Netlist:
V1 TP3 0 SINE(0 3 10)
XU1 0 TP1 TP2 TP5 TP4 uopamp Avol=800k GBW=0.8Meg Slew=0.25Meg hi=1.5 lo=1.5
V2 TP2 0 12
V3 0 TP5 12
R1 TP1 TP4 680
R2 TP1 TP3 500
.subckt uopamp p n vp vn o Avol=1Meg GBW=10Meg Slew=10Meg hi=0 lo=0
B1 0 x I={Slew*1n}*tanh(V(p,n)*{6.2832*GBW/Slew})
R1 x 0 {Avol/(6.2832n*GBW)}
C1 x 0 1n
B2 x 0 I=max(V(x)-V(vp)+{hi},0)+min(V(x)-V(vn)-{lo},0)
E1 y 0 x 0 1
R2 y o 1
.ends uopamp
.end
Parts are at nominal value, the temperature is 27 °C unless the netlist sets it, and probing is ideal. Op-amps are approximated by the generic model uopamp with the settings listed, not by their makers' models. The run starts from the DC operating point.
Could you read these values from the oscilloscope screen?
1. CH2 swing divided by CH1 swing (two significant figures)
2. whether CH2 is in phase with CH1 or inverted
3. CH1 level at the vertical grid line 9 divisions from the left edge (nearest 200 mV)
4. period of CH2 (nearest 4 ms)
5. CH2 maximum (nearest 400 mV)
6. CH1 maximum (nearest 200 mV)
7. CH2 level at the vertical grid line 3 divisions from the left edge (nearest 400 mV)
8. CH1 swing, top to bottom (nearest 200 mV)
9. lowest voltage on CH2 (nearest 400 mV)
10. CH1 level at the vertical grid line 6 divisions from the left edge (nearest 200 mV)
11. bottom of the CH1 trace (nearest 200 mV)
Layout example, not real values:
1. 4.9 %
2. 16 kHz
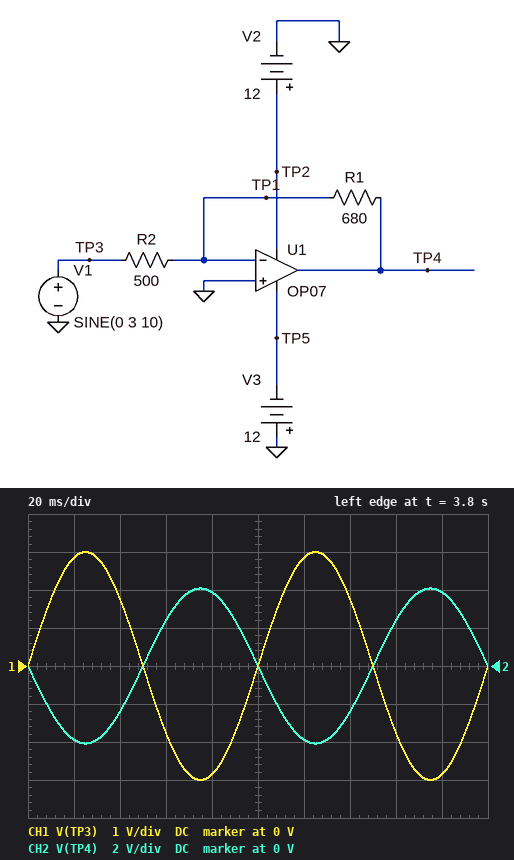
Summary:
1. 1.4
2. inverted
3. -2.8 V
4. 100 ms
5. 4.0 V
6. 3.0 V
7. 2.4 V
8. 6.0 V
9. -4.0 V
10. 2.8 V
11. -3.0 V
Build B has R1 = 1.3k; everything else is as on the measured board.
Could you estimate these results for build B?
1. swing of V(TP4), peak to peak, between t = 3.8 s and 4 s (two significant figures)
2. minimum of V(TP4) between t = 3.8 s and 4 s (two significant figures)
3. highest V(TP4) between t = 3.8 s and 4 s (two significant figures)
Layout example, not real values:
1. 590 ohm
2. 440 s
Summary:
1. 16 V
2. -7.8 V
3. 7.8 V
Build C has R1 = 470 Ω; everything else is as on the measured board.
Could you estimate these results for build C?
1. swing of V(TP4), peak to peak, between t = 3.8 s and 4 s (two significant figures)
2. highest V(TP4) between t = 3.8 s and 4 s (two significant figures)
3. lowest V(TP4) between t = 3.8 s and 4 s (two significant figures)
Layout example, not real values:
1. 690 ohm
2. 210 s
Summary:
1. 5.6 V
2. 2.8 V
3. -2.8 V
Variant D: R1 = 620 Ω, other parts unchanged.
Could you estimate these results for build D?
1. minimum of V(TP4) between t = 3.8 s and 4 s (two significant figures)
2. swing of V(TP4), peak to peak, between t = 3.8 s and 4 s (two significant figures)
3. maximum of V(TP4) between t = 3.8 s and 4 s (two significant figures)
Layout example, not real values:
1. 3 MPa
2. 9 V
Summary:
1. -3.7 V
2. 7.4 V
3. 3.7 V
